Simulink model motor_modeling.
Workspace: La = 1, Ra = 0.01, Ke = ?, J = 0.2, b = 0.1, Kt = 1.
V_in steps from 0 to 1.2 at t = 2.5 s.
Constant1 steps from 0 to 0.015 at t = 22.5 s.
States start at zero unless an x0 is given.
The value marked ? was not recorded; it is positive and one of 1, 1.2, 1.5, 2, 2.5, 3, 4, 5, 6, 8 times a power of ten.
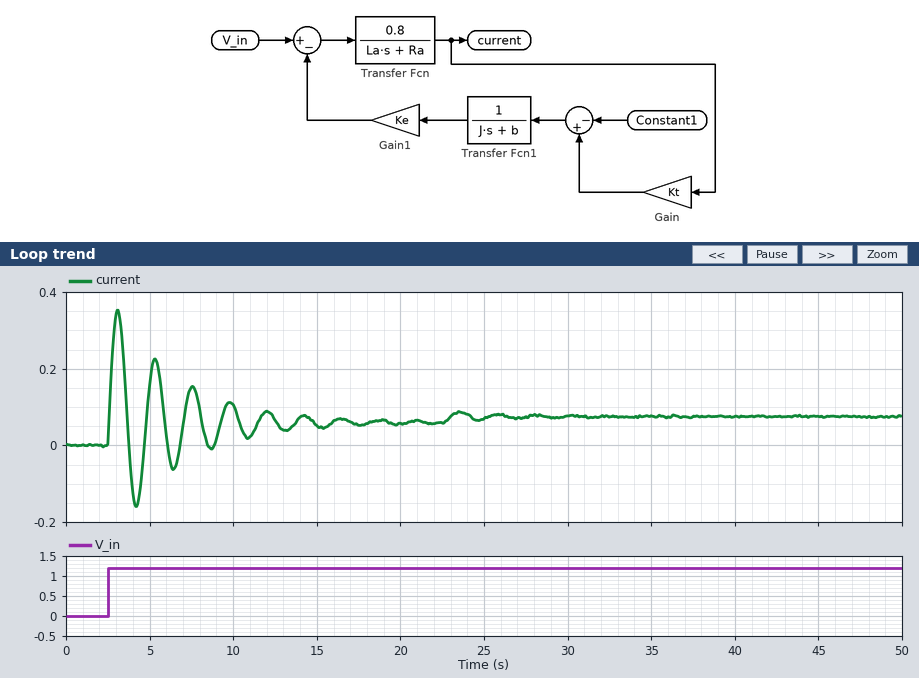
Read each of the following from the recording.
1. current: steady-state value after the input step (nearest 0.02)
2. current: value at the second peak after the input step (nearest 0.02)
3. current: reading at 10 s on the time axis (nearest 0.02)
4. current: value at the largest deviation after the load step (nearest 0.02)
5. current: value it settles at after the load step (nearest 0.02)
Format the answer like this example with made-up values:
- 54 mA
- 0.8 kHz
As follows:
- 0.06
- 0.22
- 0.10
- 0.08
- 0.08
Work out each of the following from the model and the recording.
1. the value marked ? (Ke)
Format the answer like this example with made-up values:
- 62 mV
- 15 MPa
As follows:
- 2
